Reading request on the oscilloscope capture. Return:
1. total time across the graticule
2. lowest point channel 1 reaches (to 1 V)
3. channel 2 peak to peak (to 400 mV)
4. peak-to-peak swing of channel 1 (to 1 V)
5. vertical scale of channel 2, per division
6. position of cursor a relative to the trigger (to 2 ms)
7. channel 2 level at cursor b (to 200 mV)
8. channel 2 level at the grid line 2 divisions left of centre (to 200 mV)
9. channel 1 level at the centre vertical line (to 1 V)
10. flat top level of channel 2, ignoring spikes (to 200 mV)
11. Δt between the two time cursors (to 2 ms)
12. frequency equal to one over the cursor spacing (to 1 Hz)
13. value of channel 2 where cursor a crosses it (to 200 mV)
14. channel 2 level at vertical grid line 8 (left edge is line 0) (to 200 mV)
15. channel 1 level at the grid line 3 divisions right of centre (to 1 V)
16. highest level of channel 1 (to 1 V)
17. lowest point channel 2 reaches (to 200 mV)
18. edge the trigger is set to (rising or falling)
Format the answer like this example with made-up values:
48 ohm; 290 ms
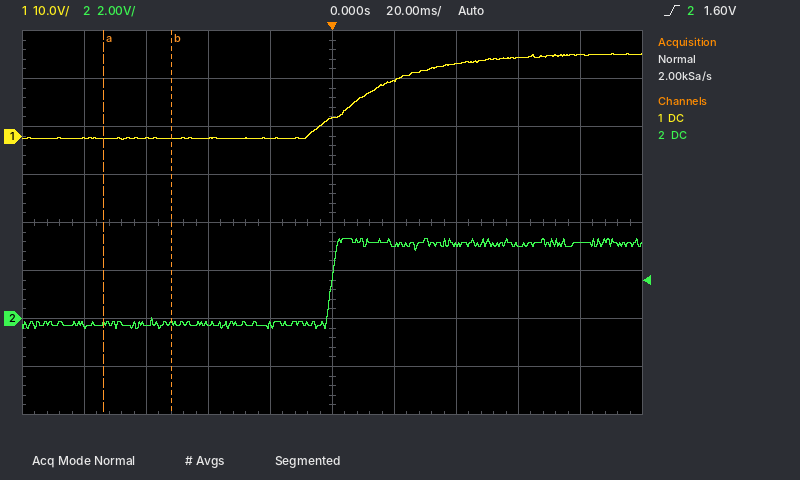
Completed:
200 ms; -1 V; 3.6 V; 18 V; 2 V; -74 ms; -200 mV; -200 mV; 4 V; 3.2 V; 22 ms; 45 Hz; -200 mV; 3.0 V; 16 V; 17 V; -400 mV; rising
